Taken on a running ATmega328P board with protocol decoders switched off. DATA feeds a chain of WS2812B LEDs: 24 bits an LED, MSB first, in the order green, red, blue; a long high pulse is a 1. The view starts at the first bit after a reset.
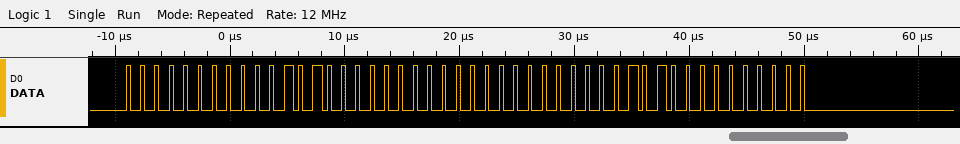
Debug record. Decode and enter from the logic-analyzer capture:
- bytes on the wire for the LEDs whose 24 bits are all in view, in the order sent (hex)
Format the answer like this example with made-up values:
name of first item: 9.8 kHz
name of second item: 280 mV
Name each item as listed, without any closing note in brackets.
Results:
bytes on the wire for the LEDs whose 24 bits are all in view, in the order sent: 00 14 00 00 14 00
